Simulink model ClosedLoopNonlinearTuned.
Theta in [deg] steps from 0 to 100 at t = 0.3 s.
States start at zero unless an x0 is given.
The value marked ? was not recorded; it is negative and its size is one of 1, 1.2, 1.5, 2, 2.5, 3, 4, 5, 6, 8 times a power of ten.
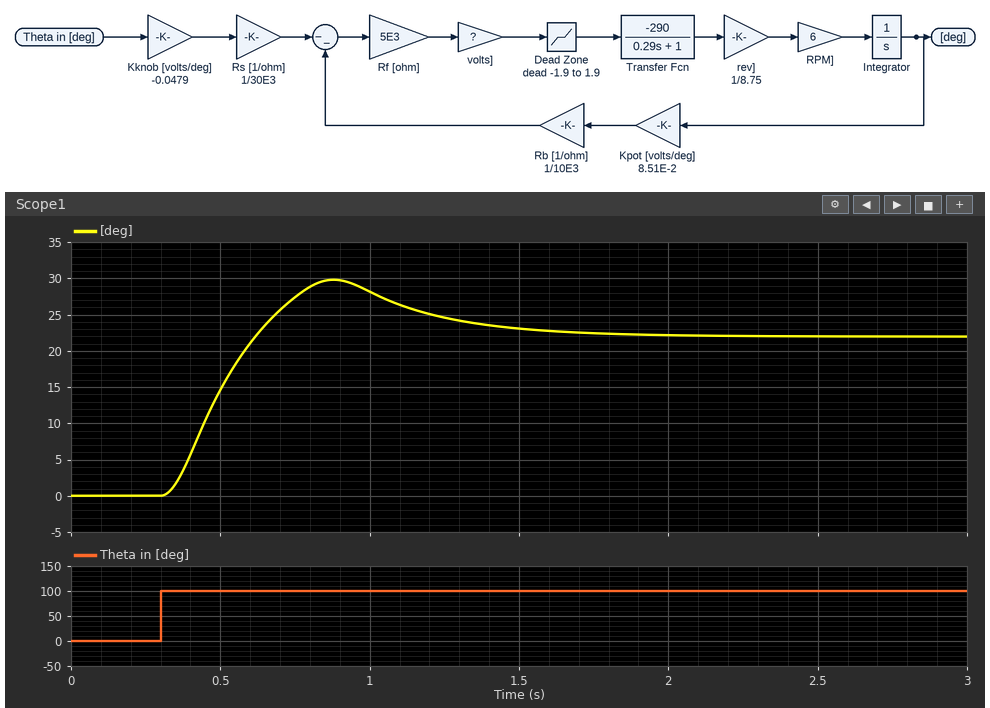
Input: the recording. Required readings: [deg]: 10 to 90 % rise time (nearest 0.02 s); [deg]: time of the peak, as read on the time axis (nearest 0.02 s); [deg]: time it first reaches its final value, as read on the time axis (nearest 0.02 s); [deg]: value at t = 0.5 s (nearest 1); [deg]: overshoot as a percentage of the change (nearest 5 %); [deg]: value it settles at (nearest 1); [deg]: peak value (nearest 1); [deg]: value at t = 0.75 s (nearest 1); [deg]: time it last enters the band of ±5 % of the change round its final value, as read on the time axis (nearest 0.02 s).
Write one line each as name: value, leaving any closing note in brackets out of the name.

[deg]: 10 to 90 % rise time: 0.22 s
[deg]: time of the peak, as read on the time axis: 0.88 s
[deg]: time it first reaches its final value, as read on the time axis: 0.62 s
[deg]: value at t = 0.5 s: 15
[deg]: overshoot as a percentage of the change: 35 %
[deg]: value it settles at: 22
[deg]: peak value: 30
[deg]: value at t = 0.75 s: 27
[deg]: time it last enters the band of ±5 % of the change round its final value, as read on the time axis: 1.50 s
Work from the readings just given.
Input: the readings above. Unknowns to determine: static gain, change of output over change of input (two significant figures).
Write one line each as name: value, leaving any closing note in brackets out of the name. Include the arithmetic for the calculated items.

static gain, change of output over change of input: (22 - 0) / (100 - 0) = 0.22
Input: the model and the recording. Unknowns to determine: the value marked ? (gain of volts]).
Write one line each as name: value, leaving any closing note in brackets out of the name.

the value marked ?: -5
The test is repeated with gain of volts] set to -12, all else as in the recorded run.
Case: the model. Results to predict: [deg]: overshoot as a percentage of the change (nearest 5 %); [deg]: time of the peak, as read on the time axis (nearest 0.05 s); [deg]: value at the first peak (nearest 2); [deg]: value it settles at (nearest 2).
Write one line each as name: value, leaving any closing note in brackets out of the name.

[deg]: overshoot as a percentage of the change: 50 %
[deg]: time of the peak, as read on the time axis: 0.50 s
[deg]: value at the first peak: 32
[deg]: value it settles at: 22
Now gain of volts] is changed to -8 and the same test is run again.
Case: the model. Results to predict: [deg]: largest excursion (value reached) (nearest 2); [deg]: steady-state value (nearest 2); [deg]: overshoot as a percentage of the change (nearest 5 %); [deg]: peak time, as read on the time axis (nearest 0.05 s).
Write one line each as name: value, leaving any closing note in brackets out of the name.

[deg]: largest excursion (value reached): 32
[deg]: steady-state value: 24
[deg]: overshoot as a percentage of the change: 35 %
[deg]: peak time, as read on the time axis: 0.60 s
